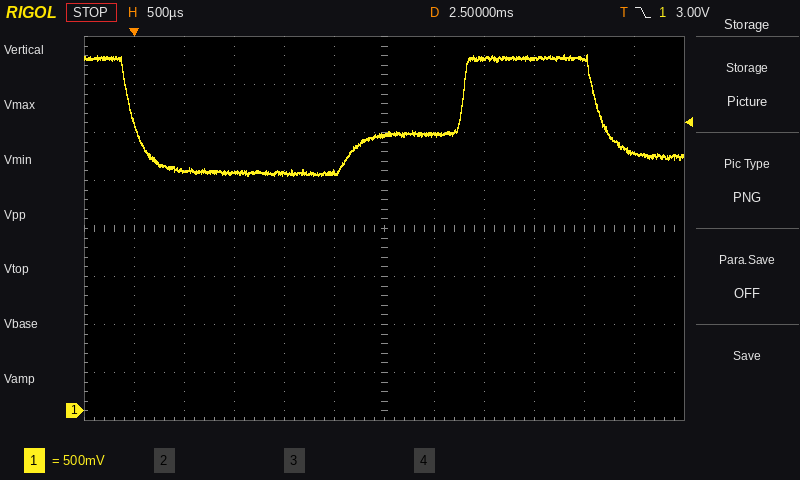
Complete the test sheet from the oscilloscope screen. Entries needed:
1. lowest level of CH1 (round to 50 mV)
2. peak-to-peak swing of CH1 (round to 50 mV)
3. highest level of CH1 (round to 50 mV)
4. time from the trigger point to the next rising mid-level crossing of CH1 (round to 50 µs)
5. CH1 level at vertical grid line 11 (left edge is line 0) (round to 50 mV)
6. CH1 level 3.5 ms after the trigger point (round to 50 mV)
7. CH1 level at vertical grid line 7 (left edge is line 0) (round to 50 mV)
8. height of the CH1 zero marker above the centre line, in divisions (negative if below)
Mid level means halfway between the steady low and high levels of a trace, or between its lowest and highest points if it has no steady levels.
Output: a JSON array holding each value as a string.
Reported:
["2.45 V", "1.25 V", "3.70 V", "3.25 ms", "2.70 V", "3.65 V", "2.90 V", "-3.8 div"]
